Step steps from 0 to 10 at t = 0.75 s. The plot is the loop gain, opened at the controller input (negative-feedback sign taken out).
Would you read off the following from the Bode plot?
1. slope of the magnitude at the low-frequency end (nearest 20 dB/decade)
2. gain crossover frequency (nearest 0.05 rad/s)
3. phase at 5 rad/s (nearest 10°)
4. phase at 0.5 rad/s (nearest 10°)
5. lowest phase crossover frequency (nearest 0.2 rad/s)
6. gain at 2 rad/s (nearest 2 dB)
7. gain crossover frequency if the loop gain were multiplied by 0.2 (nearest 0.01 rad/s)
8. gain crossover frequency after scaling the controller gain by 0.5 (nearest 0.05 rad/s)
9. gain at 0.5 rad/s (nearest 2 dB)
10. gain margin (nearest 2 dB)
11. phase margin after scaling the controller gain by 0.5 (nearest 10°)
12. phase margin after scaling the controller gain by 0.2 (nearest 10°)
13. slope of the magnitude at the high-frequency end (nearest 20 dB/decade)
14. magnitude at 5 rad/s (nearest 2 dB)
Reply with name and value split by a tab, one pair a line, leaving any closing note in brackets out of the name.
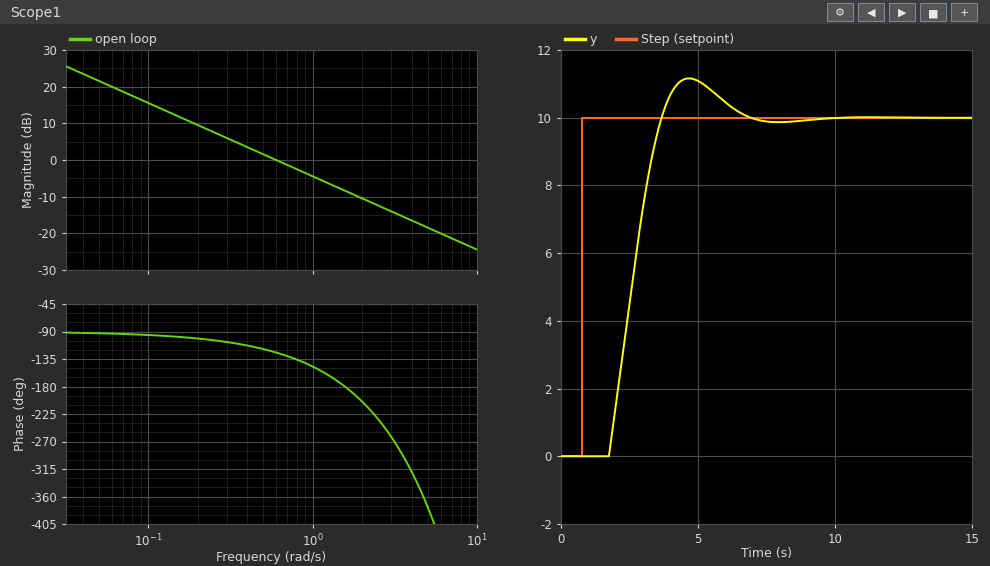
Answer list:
slope of the magnitude at the low-frequency end	-20 dB/decade
gain crossover frequency	0.60 rad/s
phase at 5 rad/s	-380°
phase at 0.5 rad/s	-120°
lowest phase crossover frequency	1.6 rad/s
gain at 2 rad/s	-10 dB
gain crossover frequency if the loop gain were multiplied by 0.2	0.12 rad/s
gain crossover frequency after scaling the controller gain by 0.5	0.30 rad/s
gain at 0.5 rad/s	2 dB
gain margin	8 dB
phase margin after scaling the controller gain by 0.5	70°
phase margin after scaling the controller gain by 0.2	80°
slope of the magnitude at the high-frequency end	-20 dB/decade
magnitude at 5 rad/s	-18 dB
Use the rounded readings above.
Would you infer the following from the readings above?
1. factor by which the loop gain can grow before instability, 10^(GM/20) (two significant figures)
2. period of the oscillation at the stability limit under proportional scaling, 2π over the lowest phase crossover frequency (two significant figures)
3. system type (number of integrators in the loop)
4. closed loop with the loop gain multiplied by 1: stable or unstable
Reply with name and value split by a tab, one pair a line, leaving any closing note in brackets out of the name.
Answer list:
factor by which the loop gain can grow before instability, 10^(GM/20)	2.5
period of the oscillation at the stability limit under proportional scaling, 2π over the lowest phase crossover frequency	3.9 s
system type	1
closed loop with the loop gain multiplied by 1: stable or unstable	stable
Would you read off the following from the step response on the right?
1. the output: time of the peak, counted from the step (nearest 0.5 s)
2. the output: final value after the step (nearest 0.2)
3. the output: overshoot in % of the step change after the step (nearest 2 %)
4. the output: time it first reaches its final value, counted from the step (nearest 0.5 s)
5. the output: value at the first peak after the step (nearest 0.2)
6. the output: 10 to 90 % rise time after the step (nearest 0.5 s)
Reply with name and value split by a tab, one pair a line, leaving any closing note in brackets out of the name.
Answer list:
the output: time of the peak, counted from the step	4.0 s
the output: final value after the step	10.0
the output: overshoot in % of the step change after the step	12 %
the output: time it first reaches its final value, counted from the step	3.0 s
the output: value at the first peak after the step	11.2
the output: 10 to 90 % rise time after the step	1.5 s
